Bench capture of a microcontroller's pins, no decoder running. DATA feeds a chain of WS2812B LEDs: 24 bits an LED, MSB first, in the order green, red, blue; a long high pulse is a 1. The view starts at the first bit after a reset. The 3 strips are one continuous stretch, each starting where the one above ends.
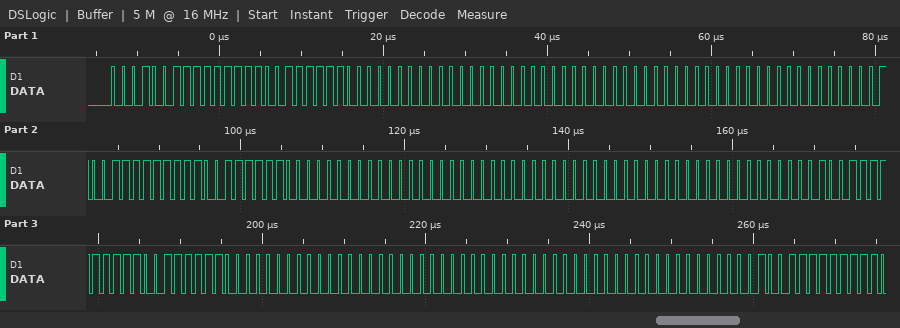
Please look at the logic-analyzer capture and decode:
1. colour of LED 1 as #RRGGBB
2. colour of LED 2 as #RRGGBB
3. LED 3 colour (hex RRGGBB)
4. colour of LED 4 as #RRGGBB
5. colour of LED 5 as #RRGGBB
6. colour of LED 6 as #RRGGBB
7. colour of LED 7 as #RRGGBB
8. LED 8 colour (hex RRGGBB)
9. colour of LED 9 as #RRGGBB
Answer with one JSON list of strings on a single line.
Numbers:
["#FE137E", "#000000", "#000000", "#FE137E", "#000000", "#000000", "#FE137E", "#000000", "#000000"]
